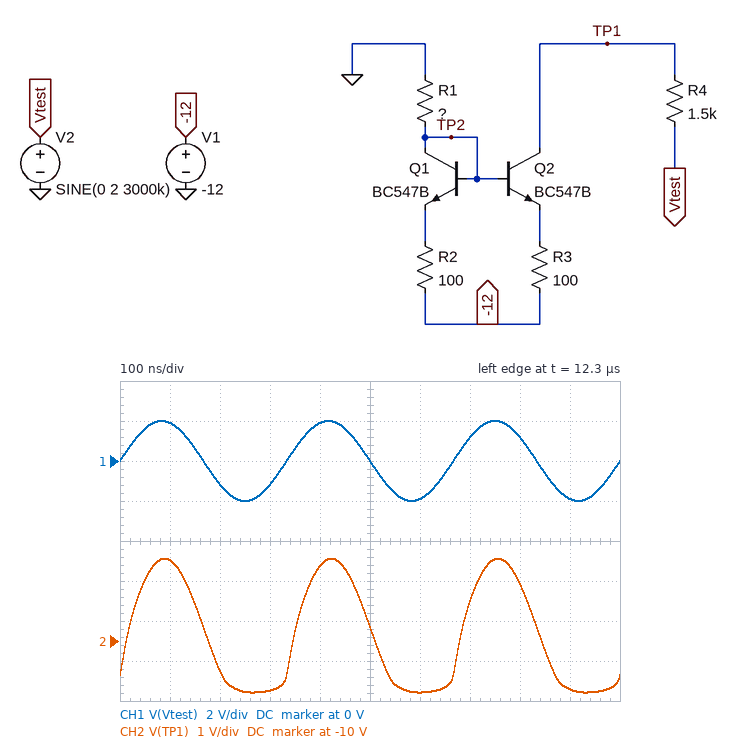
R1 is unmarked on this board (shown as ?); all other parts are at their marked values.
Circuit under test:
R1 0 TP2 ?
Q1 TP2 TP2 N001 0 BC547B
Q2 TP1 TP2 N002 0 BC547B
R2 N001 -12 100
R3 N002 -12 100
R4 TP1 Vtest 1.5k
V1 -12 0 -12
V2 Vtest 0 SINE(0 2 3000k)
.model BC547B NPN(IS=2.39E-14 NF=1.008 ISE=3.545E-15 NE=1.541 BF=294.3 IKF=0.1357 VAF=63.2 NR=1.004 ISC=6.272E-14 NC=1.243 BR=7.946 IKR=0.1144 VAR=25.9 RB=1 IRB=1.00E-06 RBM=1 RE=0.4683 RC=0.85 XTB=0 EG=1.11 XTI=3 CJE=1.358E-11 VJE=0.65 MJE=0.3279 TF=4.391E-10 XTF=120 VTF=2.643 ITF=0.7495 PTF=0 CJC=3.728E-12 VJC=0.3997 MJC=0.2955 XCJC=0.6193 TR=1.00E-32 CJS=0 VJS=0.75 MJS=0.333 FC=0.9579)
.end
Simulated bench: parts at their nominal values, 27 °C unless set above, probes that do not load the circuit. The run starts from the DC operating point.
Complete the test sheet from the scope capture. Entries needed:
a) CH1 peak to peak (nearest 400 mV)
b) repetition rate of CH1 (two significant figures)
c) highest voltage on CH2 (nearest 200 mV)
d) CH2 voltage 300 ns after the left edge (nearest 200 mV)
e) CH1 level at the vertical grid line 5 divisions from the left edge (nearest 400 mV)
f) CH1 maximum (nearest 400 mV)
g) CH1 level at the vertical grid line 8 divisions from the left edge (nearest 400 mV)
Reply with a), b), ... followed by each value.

a) 4.0 V
b) 3.0 MHz
c) -8.0 V
d) -11.2 V
e) 0 V
f) 2.0 V
g) 1.2 V
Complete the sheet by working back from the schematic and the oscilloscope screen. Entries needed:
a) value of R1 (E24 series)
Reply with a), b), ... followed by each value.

a) 1.6 kΩ
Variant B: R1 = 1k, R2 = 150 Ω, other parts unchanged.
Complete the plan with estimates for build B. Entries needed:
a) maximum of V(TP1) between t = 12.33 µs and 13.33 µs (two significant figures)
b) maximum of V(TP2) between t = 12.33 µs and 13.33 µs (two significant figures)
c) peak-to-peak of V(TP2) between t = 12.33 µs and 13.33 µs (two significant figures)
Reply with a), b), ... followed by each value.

a) -11 V
b) -10 V
c) 140 mV
